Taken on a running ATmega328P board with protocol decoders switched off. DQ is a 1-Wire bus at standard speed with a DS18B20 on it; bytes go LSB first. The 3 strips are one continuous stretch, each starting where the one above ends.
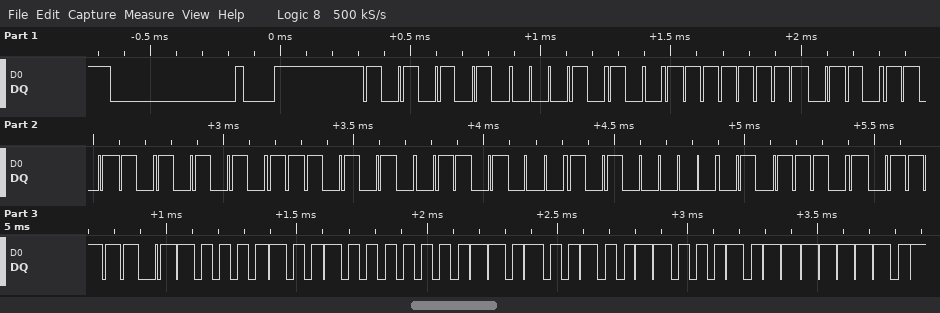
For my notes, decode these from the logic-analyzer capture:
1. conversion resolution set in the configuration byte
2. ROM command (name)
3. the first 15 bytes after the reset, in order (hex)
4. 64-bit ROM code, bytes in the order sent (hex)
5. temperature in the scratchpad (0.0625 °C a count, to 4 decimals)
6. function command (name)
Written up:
12 bits
Match ROM
55 28 FF B6 55 57 16 05 BA BE 21 01 4B 46 7F
28 FF B6 55 57 16 05 BA
18.0625 °C
Read Scratchpad
